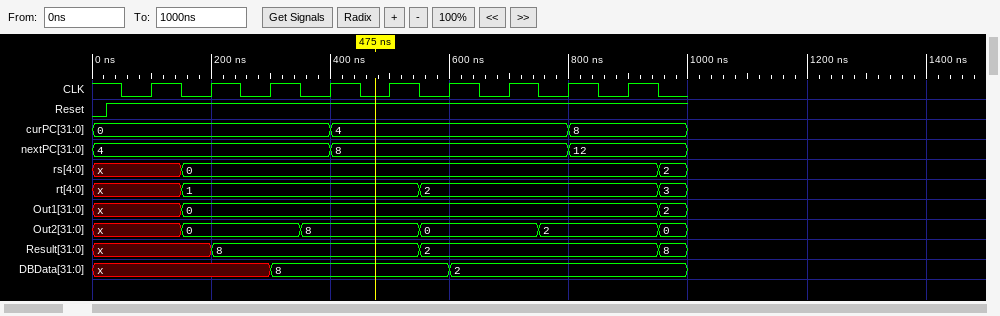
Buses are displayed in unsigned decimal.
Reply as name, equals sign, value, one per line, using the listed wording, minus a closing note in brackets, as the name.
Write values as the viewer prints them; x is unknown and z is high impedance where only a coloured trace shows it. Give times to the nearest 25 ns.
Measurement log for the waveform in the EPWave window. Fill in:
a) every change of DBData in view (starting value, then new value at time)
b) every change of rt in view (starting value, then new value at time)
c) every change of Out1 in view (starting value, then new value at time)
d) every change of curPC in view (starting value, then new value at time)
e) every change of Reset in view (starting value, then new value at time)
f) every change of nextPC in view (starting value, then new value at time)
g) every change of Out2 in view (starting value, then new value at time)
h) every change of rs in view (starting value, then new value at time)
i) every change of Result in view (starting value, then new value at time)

every change of DBData in view = x, 8 at 300 ns, 2 at 600 ns
every change of rt in view = x, 1 at 150 ns, 2 at 550 ns, 3 at 950 ns
every change of Out1 in view = x, 0 at 150 ns, 2 at 950 ns
every change of curPC in view = 0, 4 at 400 ns, 8 at 800 ns
every change of Reset in view = 0, 1 at 25 ns
every change of nextPC in view = 4, 8 at 400 ns, 12 at 800 ns
every change of Out2 in view = x, 0 at 150 ns, 8 at 350 ns, 0 at 550 ns, 2 at 750 ns, 0 at 950 ns
every change of rs in view = x, 0 at 150 ns, 2 at 950 ns
every change of Result in view = x, 8 at 200 ns, 2 at 550 ns, 8 at 950 ns
